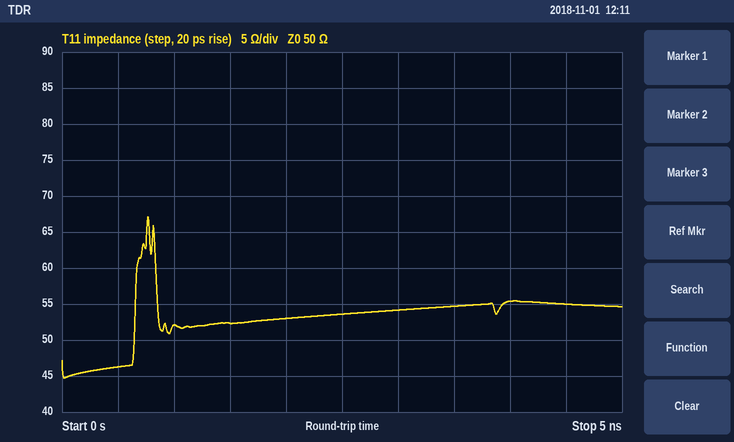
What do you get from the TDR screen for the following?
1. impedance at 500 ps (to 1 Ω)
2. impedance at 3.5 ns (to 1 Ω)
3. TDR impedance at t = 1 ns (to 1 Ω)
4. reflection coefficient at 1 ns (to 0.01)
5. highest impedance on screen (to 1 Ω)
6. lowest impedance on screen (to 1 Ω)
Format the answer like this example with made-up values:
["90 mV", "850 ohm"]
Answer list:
["46 Ω", "55 Ω", "52 Ω", "+0.02", "67 Ω", "45 Ω"]
